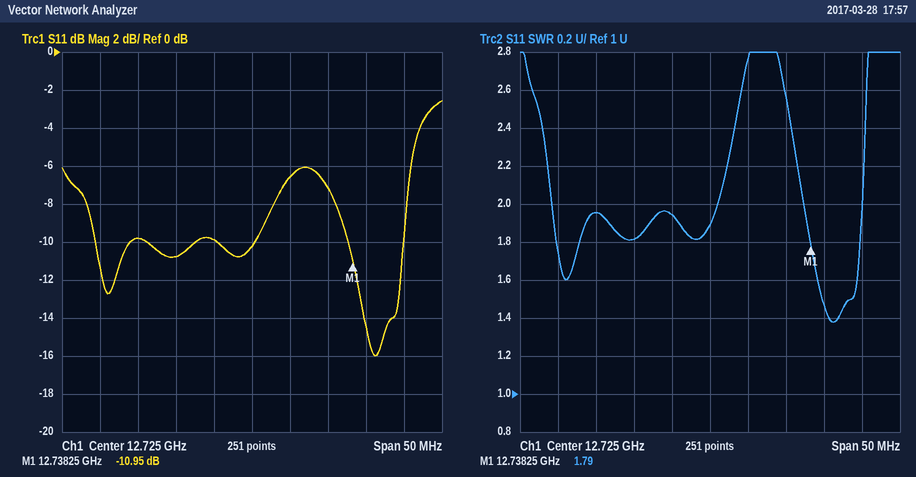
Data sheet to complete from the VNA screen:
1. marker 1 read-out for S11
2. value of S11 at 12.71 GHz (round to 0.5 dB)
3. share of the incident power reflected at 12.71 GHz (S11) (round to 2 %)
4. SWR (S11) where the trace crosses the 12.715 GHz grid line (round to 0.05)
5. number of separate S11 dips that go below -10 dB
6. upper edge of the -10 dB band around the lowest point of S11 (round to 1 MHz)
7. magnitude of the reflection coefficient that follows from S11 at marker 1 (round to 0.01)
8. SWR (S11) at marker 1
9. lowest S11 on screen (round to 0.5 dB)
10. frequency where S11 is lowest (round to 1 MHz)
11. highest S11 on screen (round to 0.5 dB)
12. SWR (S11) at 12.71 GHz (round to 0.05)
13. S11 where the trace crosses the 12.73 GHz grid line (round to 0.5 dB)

-10.95 dB
-10.0 dB
10 %
1.80
2
12.745 GHz
0.28
1.79
-16.0 dB
12.741 GHz
-2.5 dB
1.95
-6.5 dB
